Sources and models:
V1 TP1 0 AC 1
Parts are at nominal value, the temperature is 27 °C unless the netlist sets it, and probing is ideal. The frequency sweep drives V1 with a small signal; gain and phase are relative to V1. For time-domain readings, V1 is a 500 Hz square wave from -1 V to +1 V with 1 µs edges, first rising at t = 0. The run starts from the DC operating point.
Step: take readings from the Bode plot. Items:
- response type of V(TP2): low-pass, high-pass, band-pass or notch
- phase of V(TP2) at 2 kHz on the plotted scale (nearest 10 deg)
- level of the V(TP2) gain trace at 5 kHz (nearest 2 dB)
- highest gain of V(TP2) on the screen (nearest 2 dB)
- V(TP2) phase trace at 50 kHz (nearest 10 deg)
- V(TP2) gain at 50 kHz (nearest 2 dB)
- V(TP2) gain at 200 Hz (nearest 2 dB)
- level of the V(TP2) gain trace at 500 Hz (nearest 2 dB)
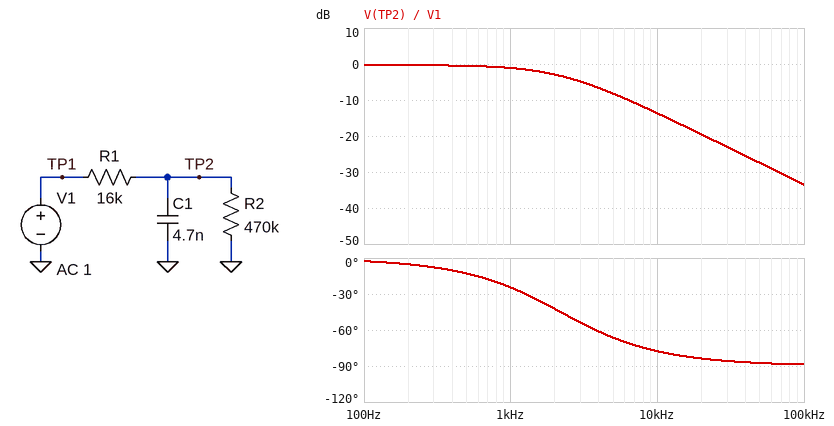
low-pass
-40 deg
-8 dB
0 dB
-90 deg
-28 dB
0 dB
0 dB
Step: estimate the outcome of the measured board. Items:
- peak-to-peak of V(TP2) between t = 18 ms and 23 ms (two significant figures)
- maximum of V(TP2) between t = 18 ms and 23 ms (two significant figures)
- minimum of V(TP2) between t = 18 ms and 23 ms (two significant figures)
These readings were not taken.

1.9 V
970 mV
-970 mV
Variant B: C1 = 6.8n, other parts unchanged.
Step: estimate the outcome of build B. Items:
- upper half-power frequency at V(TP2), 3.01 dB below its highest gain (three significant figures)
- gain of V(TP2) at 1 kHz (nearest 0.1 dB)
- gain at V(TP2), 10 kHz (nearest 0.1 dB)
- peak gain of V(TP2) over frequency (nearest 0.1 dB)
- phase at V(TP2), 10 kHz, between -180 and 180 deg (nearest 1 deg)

1.51 kHz
-1.9 dB
-16.8 dB
-0.3 dB
-81 deg
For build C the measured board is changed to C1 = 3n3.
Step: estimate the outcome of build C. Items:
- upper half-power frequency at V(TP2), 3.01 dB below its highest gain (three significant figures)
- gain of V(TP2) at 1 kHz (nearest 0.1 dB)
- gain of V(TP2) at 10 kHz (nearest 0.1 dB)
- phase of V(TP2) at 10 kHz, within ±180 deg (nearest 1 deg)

3.12 kHz
-0.7 dB
-10.8 dB
-73 deg
